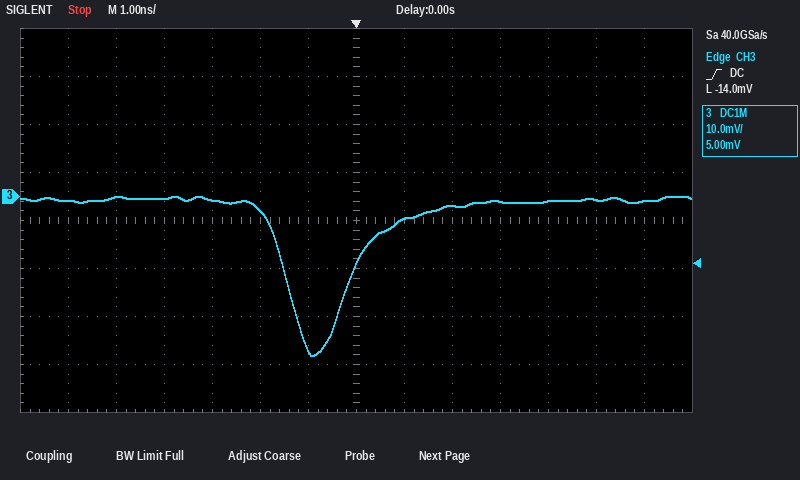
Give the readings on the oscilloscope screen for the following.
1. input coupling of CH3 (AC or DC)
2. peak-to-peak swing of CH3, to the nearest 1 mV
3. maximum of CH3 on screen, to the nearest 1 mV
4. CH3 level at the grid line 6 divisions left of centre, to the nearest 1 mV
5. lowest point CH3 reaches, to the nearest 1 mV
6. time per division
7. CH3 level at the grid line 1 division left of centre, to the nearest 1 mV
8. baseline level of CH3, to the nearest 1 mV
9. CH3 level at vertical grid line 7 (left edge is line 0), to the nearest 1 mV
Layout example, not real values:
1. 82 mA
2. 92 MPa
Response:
1. DC
2. 33 mV
3. 0 mV
4. -1 mV
5. -33 mV
6. 1 ns
7. -32 mV
8. -1 mV
9. -14 mV
